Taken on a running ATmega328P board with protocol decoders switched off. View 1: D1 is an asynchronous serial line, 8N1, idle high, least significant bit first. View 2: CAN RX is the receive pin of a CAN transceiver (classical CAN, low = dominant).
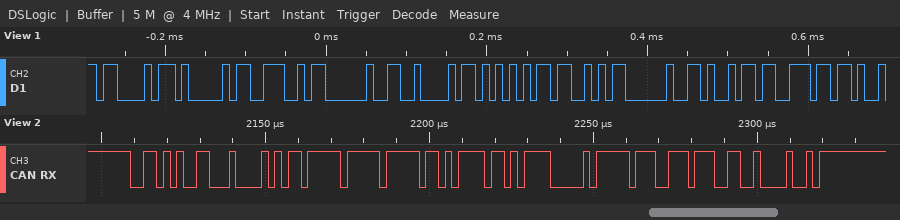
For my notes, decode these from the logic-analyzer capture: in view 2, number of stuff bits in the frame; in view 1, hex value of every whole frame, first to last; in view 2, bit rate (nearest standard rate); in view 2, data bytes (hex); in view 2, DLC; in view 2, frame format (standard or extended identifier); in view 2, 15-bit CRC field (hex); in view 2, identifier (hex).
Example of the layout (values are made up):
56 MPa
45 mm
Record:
5
0x43 0x41 0x4E 0x20 0x42 0x55 0x53 0x20 0x69 0x6E
500 kbit/s
56 FF FF AF 6B C0 FF 3B
8
standard
0x4C84
0x353
